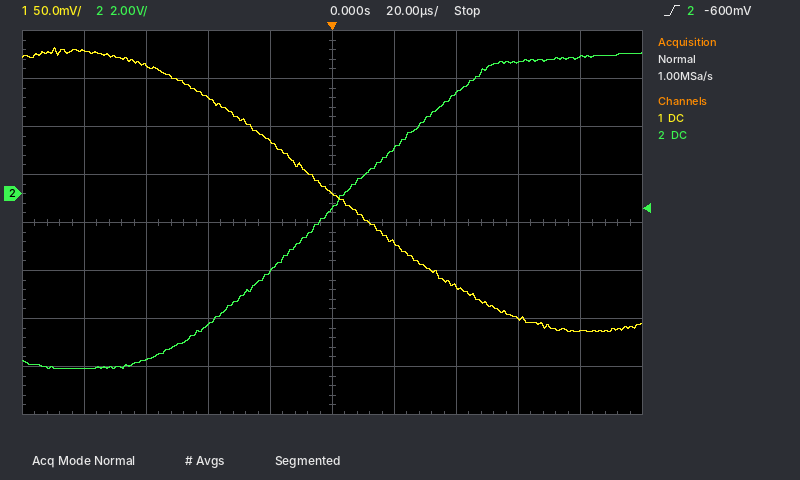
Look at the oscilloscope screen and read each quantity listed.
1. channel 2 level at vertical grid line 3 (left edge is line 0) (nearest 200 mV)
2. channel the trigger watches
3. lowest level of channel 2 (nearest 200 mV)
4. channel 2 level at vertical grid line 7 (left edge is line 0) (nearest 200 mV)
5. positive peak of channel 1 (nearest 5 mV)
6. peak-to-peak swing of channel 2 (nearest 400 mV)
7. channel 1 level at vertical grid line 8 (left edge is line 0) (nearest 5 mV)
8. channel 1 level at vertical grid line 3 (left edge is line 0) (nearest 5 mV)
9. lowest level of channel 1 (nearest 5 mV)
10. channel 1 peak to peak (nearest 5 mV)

-5.4 V
channel 2
-7.2 V
4.2 V
150 mV
13.2 V
-130 mV
100 mV
-145 mV
295 mV
